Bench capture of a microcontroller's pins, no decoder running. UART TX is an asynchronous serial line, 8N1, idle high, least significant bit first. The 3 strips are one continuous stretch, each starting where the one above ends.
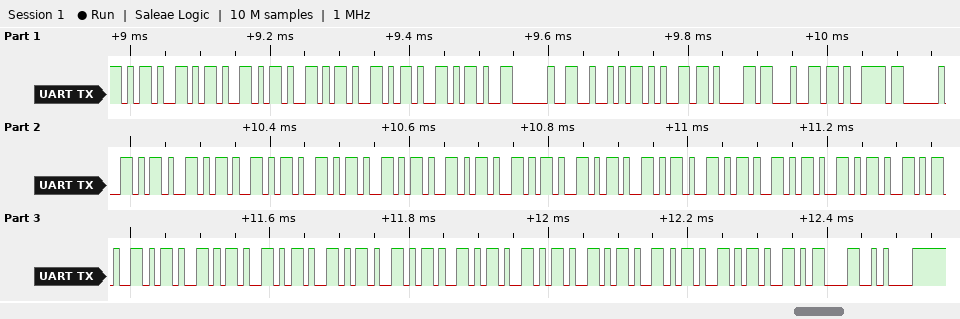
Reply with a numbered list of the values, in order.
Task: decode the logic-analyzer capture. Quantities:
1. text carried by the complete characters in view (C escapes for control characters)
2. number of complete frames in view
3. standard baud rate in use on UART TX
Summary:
1. "------ Ready -----------------------\r\n"
2. 38
3. 115200 baud
